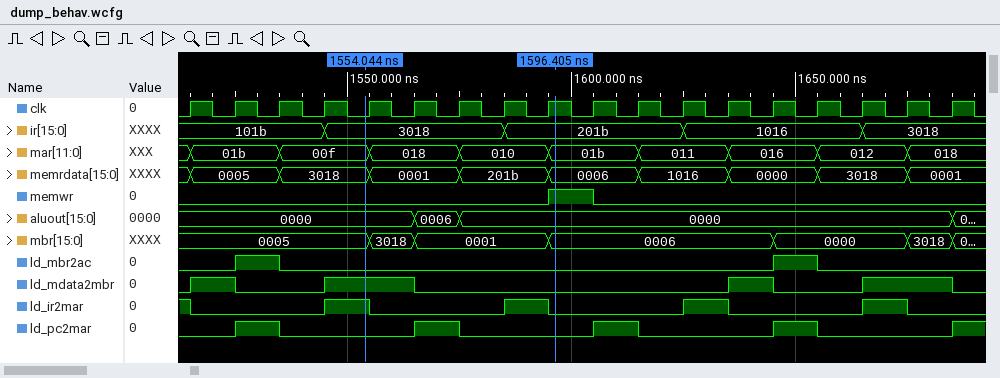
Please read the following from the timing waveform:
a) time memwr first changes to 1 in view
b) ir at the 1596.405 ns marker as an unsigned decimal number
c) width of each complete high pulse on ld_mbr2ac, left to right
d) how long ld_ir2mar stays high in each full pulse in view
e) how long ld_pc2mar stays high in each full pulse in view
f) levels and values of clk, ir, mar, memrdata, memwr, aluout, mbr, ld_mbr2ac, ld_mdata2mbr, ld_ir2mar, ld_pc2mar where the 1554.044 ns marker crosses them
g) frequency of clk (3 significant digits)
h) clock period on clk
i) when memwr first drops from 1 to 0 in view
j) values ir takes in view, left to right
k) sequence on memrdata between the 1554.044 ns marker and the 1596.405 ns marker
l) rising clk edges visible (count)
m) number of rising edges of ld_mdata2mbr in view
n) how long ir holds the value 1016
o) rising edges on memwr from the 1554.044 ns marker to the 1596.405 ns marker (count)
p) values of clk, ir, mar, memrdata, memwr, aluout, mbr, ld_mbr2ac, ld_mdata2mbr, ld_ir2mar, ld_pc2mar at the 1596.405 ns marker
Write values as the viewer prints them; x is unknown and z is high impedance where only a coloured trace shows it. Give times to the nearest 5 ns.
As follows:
1595 ns
8219
10 ns, 10 ns
10 ns, 10 ns, 10 ns, 10 ns
10 ns, 10 ns, 10 ns, 10 ns
clk=0, ir=3018, mar=00f, memrdata=3018, memwr=0, aluout=0000, mbr=0005, ld_mbr2ac=0, ld_mdata2mbr=1, ld_ir2mar=1, ld_pc2mar=0
100 MHz
10 ns
1605 ns
101b, 3018, 201b, 1016, 3018
3018, 0001, 201b, 0006
18
4
40 ns
1
clk=1, ir=201b, mar=01b, memrdata=0006, memwr=1, aluout=0000, mbr=0006, ld_mbr2ac=0, ld_mdata2mbr=0, ld_ir2mar=0, ld_pc2mar=0
